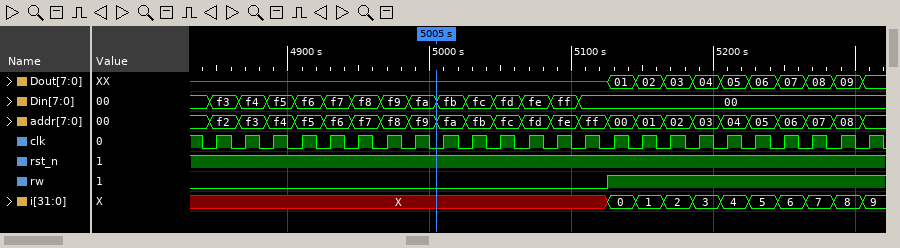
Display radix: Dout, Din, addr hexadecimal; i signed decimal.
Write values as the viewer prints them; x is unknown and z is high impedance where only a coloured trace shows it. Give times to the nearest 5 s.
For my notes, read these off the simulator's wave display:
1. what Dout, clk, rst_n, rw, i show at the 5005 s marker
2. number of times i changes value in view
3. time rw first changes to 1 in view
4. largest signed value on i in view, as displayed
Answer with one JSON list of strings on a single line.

["Dout=z, clk=0, rst_n=1, rw=0, i=X", "10", "5125 s", "9"]
